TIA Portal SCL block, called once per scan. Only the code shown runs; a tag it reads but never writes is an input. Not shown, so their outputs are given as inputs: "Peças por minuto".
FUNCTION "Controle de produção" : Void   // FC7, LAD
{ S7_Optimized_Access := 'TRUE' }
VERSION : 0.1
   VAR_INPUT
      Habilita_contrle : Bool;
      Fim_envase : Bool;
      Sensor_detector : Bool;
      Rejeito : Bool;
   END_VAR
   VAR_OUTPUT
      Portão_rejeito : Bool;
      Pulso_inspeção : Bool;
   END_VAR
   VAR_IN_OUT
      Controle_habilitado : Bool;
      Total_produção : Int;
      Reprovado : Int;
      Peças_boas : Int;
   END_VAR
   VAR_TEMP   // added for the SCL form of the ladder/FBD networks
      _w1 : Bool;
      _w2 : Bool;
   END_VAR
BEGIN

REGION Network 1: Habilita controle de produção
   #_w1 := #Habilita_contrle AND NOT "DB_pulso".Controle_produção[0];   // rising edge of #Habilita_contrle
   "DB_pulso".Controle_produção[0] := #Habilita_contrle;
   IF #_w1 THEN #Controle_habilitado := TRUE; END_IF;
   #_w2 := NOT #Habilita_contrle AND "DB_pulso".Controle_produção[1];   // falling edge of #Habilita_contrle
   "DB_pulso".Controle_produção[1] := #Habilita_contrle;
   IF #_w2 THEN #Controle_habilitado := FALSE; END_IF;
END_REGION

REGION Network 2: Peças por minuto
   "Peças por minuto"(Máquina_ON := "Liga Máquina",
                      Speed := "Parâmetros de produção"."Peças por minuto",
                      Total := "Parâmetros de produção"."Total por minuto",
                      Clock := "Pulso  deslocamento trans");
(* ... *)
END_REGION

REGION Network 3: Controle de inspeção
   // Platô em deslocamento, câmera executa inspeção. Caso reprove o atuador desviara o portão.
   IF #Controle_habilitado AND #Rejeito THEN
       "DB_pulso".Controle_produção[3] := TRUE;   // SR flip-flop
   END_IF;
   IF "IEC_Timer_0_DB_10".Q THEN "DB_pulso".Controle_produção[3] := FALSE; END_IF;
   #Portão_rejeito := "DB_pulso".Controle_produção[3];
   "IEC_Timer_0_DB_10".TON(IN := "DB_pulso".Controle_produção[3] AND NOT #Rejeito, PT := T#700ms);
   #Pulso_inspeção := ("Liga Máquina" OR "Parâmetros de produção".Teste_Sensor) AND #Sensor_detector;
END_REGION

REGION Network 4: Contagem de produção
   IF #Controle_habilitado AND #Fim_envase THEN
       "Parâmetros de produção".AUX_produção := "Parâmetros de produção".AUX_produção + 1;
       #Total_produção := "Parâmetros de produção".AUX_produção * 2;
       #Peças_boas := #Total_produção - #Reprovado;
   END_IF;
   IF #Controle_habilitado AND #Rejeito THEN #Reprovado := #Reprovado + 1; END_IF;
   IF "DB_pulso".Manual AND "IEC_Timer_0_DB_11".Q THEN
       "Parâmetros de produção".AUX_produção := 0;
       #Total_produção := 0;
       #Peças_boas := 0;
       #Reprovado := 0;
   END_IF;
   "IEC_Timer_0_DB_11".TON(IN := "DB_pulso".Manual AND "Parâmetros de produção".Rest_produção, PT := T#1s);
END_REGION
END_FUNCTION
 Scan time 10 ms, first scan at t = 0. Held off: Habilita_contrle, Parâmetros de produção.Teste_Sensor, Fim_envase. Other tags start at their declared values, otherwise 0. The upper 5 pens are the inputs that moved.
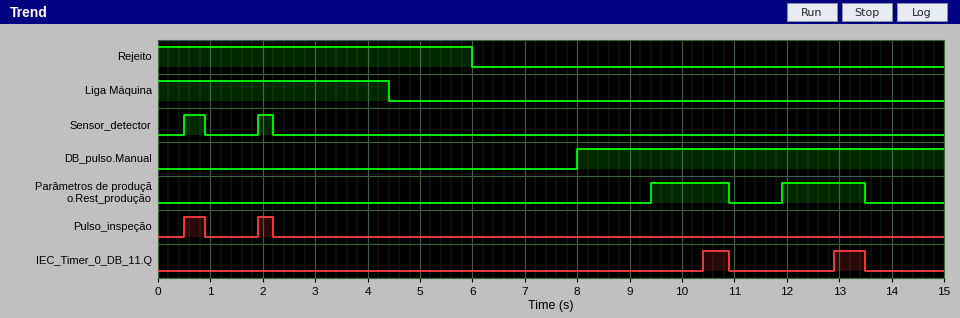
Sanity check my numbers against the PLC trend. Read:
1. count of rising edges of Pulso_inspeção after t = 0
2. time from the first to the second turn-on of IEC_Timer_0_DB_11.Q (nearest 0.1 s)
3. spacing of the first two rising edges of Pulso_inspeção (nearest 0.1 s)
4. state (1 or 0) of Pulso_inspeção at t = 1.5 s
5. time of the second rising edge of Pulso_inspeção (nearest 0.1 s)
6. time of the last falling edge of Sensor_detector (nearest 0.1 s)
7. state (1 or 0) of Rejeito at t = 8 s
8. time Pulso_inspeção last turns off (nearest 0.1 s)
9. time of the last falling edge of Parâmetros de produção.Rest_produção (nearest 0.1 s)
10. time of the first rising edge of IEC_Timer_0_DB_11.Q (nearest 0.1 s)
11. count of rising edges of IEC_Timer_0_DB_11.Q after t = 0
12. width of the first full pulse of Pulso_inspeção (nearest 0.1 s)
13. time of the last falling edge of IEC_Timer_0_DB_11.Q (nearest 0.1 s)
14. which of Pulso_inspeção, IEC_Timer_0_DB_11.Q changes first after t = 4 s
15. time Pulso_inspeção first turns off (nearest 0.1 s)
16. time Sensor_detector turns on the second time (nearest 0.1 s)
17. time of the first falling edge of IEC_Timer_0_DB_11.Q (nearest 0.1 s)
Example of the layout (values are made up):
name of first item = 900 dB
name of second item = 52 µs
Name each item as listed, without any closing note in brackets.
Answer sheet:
count of rising edges of Pulso_inspeção after t = 0 = 2
time from the first to the second turn-on of IEC_Timer_0_DB_11.Q = 2.5 s
spacing of the first two rising edges of Pulso_inspeção = 1.4 s
state (1 or 0) of Pulso_inspeção at t = 1.5 s = 0
time of the second rising edge of Pulso_inspeção = 1.9 s
time of the last falling edge of Sensor_detector = 2.2 s
state (1 or 0) of Rejeito at t = 8 s = 0
time Pulso_inspeção last turns off = 2.2 s
time of the last falling edge of Parâmetros de produção.Rest_produção = 13.5 s
time of the first rising edge of IEC_Timer_0_DB_11.Q = 10.4 s
count of rising edges of IEC_Timer_0_DB_11.Q after t = 0 = 2
width of the first full pulse of Pulso_inspeção = 0.4 s
time of the last falling edge of IEC_Timer_0_DB_11.Q = 13.5 s
which of Pulso_inspeção, IEC_Timer_0_DB_11.Q changes first after t = 4 s = IEC_Timer_0_DB_11.Q
time Pulso_inspeção first turns off = 0.9 s
time Sensor_detector turns on the second time = 1.9 s
time of the first falling edge of IEC_Timer_0_DB_11.Q = 10.9 s
